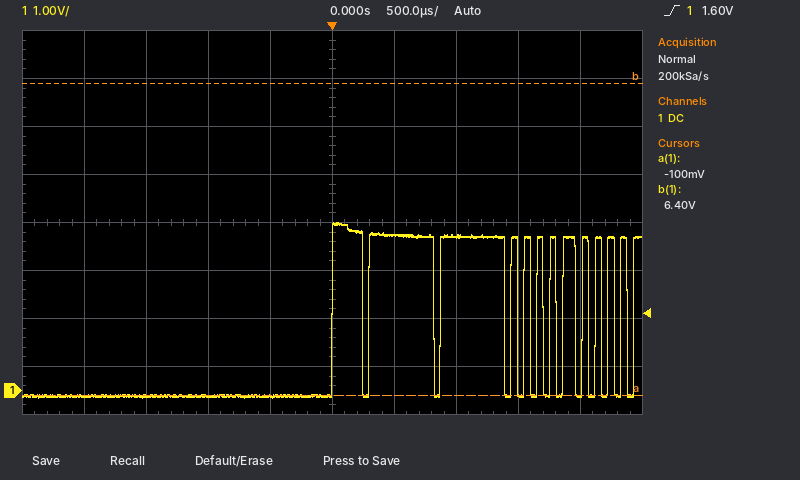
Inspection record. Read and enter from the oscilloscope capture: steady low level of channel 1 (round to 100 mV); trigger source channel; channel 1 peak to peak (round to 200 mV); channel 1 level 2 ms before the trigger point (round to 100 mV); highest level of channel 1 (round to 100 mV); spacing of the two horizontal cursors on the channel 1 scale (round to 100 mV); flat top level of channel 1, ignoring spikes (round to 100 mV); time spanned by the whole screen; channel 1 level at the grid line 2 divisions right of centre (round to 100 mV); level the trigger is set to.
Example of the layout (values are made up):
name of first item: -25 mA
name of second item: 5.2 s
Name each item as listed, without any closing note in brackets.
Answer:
steady low level of channel 1: -100 mV
trigger source channel: channel 1
channel 1 peak to peak: 3.6 V
channel 1 level 2 ms before the trigger point: -100 mV
highest level of channel 1: 3.5 V
spacing of the two horizontal cursors on the channel 1 scale: 6.5 V
flat top level of channel 1, ignoring spikes: 3.2 V
time spanned by the whole screen: 5 ms
channel 1 level at the grid line 2 divisions right of centre: 3.2 V
level the trigger is set to: 1.60 V
